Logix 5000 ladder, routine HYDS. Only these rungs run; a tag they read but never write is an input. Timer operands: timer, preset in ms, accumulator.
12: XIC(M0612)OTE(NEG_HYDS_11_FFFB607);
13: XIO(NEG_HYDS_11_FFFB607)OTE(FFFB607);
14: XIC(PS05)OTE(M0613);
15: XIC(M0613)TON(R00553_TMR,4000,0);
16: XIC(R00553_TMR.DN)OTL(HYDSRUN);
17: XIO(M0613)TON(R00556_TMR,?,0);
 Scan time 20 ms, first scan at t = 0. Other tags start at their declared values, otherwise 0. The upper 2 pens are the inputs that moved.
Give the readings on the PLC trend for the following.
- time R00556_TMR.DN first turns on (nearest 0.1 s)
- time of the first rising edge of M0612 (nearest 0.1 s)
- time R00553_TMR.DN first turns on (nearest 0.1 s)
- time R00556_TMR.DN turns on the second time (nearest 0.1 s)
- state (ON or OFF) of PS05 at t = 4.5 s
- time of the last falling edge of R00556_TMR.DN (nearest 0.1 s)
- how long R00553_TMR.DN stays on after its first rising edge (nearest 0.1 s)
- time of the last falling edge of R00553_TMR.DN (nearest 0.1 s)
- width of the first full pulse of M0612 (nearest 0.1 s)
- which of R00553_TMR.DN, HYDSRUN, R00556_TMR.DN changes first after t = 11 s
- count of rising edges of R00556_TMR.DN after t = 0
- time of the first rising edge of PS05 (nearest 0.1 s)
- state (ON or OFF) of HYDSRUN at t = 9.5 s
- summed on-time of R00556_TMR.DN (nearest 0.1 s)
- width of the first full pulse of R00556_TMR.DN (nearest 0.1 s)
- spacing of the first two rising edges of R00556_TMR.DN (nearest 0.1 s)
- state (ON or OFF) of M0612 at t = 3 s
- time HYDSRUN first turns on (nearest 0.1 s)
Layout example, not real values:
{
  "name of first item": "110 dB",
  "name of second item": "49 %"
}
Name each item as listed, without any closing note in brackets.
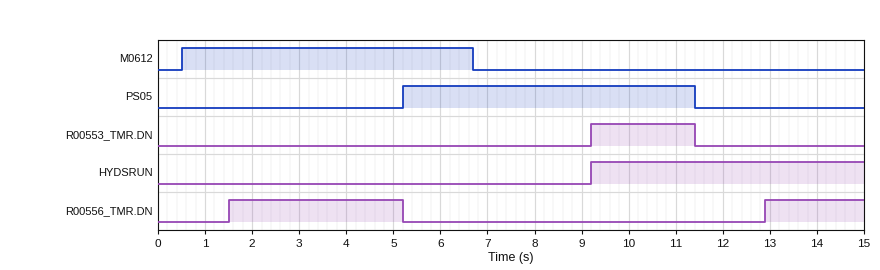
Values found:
{
  "time R00556_TMR.DN first turns on": "1.5 s",
  "time of the first rising edge of M0612": "0.5 s",
  "time R00553_TMR.DN first turns on": "9.2 s",
  "time R00556_TMR.DN turns on the second time": "12.9 s",
  "state (ON or OFF) of PS05 at t = 4.5 s": "OFF",
  "time of the last falling edge of R00556_TMR.DN": "5.2 s",
  "how long R00553_TMR.DN stays on after its first rising edge": "2.2 s",
  "time of the last falling edge of R00553_TMR.DN": "11.4 s",
  "width of the first full pulse of M0612": "6.2 s",
  "which of R00553_TMR.DN, HYDSRUN, R00556_TMR.DN changes first after t = 11 s": "R00553_TMR.DN",
  "count of rising edges of R00556_TMR.DN after t = 0": "2",
  "time of the first rising edge of PS05": "5.2 s",
  "state (ON or OFF) of HYDSRUN at t = 9.5 s": "ON",
  "summed on-time of R00556_TMR.DN": "5.8 s",
  "width of the first full pulse of R00556_TMR.DN": "3.7 s",
  "spacing of the first two rising edges of R00556_TMR.DN": "11.4 s",
  "state (ON or OFF) of M0612 at t = 3 s": "ON",
  "time HYDSRUN first turns on": "9.2 s"
}
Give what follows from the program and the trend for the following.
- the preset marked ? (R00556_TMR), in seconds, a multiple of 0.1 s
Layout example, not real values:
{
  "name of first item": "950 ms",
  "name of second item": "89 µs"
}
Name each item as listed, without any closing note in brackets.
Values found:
{
  "the preset marked ? (R00556_TMR), in seconds, a multiple of 0.1 s": "1.5 s"
}
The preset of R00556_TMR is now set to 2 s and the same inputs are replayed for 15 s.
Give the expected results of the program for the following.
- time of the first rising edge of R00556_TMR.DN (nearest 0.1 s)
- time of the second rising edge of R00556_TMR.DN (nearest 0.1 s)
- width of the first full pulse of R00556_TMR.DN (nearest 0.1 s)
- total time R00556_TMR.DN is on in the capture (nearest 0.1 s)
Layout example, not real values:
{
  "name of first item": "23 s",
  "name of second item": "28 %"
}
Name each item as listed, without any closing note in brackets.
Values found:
{
  "time of the first rising edge of R00556_TMR.DN": "2.0 s",
  "time of the second rising edge of R00556_TMR.DN": "13.4 s",
  "width of the first full pulse of R00556_TMR.DN": "3.2 s",
  "total time R00556_TMR.DN is on in the capture": "4.8 s"
}
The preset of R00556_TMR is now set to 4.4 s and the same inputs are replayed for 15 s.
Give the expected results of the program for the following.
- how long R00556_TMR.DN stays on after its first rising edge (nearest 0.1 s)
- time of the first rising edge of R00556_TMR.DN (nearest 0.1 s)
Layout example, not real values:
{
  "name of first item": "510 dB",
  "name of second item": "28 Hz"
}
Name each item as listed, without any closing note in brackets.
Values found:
{
  "how long R00556_TMR.DN stays on after its first rising edge": "0.8 s",
  "time of the first rising edge of R00556_TMR.DN": "4.4 s"
}
